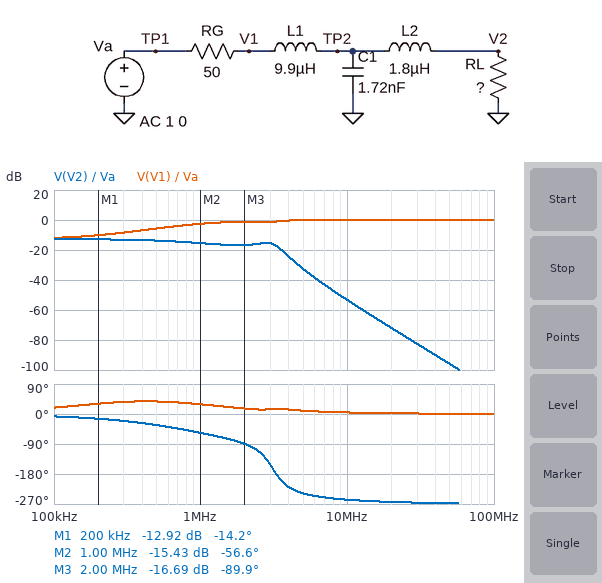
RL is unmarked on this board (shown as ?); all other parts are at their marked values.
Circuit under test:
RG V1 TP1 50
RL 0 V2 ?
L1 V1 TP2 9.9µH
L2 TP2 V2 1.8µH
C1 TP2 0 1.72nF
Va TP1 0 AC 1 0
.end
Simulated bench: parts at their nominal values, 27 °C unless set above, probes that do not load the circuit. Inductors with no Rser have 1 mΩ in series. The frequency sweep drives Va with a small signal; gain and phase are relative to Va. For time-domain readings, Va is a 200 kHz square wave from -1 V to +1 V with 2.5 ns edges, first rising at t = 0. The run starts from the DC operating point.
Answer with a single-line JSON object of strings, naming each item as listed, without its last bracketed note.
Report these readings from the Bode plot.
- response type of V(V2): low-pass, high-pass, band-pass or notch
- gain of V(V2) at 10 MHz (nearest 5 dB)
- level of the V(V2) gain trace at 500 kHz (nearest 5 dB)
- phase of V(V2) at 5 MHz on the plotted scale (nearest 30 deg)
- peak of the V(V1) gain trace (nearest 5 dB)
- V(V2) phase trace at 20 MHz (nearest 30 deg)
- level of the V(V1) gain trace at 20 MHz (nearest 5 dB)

{"response type of V(V2): low-pass, high-pass, band-pass or notch": "low-pass", "gain of V(V2) at 10 MHz": "-55 dB", "level of the V(V2) gain trace at 500 kHz": "-15 dB", "phase of V(V2) at 5 MHz on the plotted scale": "-240 deg", "peak of the V(V1) gain trace": "0 dB", "V(V2) phase trace at 20 MHz": "-270 deg", "level of the V(V1) gain trace at 20 MHz": "0 dB"}
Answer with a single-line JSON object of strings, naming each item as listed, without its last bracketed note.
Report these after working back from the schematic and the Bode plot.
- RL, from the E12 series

{"RL, from the E12 series": "15 Ω"}
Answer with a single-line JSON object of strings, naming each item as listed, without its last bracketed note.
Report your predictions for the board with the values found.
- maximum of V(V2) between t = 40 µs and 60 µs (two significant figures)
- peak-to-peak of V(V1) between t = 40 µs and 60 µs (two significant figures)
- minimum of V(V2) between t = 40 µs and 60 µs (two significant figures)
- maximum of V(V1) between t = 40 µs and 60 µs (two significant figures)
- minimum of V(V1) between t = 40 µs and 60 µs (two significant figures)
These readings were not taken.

{"maximum of V(V2) between t = 40 µs and 60 µs": "230 mV", "peak-to-peak of V(V1) between t = 40 µs and 60 µs": "3.5 V", "minimum of V(V2) between t = 40 µs and 60 µs": "-230 mV", "maximum of V(V1) between t = 40 µs and 60 µs": "1.8 V", "minimum of V(V1) between t = 40 µs and 60 µs": "-1.8 V"}
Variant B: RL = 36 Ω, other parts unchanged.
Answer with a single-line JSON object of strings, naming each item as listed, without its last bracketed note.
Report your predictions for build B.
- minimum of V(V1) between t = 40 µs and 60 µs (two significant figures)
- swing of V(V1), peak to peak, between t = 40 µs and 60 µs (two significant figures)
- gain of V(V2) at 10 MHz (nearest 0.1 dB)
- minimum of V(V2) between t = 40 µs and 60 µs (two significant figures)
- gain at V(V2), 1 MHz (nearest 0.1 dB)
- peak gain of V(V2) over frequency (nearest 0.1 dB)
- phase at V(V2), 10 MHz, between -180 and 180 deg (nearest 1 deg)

{"minimum of V(V1) between t = 40 µs and 60 µs": "-1.6 V", "swing of V(V1), peak to peak, between t = 40 µs and 60 µs": "3.1 V", "gain of V(V2) at 10 MHz": "-46.1 dB", "minimum of V(V2) between t = 40 µs and 60 µs": "-420 mV", "gain at V(V2), 1 MHz": "-9.0 dB", "peak gain of V(V2) over frequency": "-7.6 dB", "phase at V(V2), 10 MHz, between -180 and 180 deg": "114 deg"}
